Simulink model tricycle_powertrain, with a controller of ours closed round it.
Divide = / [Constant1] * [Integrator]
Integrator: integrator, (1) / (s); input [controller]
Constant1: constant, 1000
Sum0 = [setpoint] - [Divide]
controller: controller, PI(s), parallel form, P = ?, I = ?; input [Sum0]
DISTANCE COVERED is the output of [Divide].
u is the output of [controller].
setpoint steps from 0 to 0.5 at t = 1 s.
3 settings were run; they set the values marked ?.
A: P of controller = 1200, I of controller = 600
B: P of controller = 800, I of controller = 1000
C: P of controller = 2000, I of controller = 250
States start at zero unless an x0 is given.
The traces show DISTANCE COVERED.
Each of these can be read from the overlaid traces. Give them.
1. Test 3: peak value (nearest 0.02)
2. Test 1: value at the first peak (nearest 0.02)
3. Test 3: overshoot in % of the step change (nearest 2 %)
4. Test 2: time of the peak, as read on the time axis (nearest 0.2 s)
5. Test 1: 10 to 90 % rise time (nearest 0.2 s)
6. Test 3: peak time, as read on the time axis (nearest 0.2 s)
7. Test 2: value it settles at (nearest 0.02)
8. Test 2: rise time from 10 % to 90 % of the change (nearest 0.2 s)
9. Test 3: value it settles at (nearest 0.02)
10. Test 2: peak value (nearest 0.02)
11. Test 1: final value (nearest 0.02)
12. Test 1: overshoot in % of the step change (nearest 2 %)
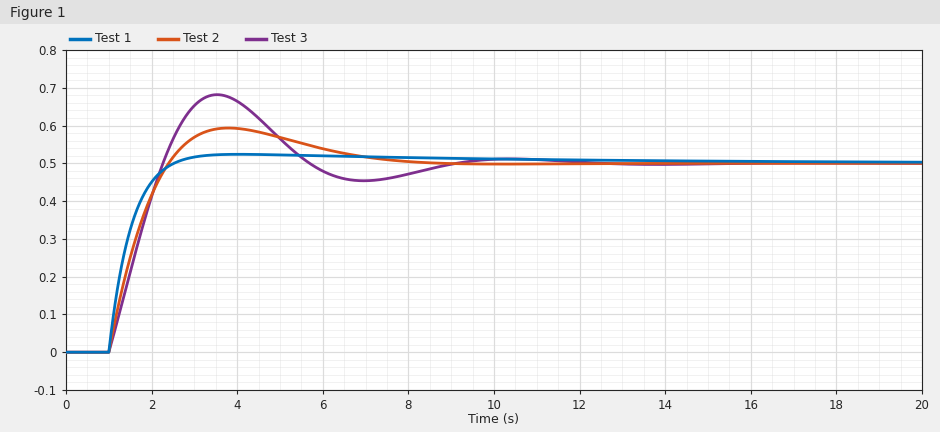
0.68
0.52
36 %
3.8 s
1.0 s
3.6 s
0.50
1.0 s
0.50
0.60
0.50
4 %
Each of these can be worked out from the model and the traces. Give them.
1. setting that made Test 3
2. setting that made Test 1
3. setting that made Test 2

B
C
A
